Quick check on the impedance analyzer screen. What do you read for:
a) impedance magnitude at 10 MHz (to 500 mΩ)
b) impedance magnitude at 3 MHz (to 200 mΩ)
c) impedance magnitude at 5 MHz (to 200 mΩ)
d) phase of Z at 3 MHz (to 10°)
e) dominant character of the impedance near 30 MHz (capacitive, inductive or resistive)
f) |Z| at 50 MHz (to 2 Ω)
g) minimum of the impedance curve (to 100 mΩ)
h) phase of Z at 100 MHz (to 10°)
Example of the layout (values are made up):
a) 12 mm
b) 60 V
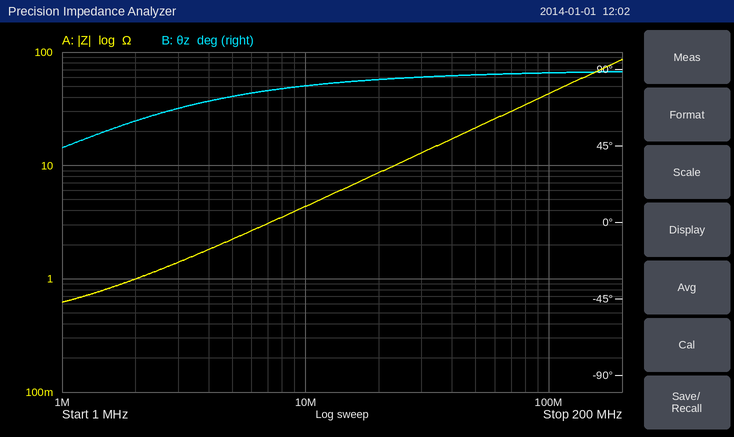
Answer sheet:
a) 4.5 Ω
b) 1.4 Ω
c) 2.2 Ω
d) 70°
e) inductive
f) 22 Ω
g) 600 mΩ
h) 90°
